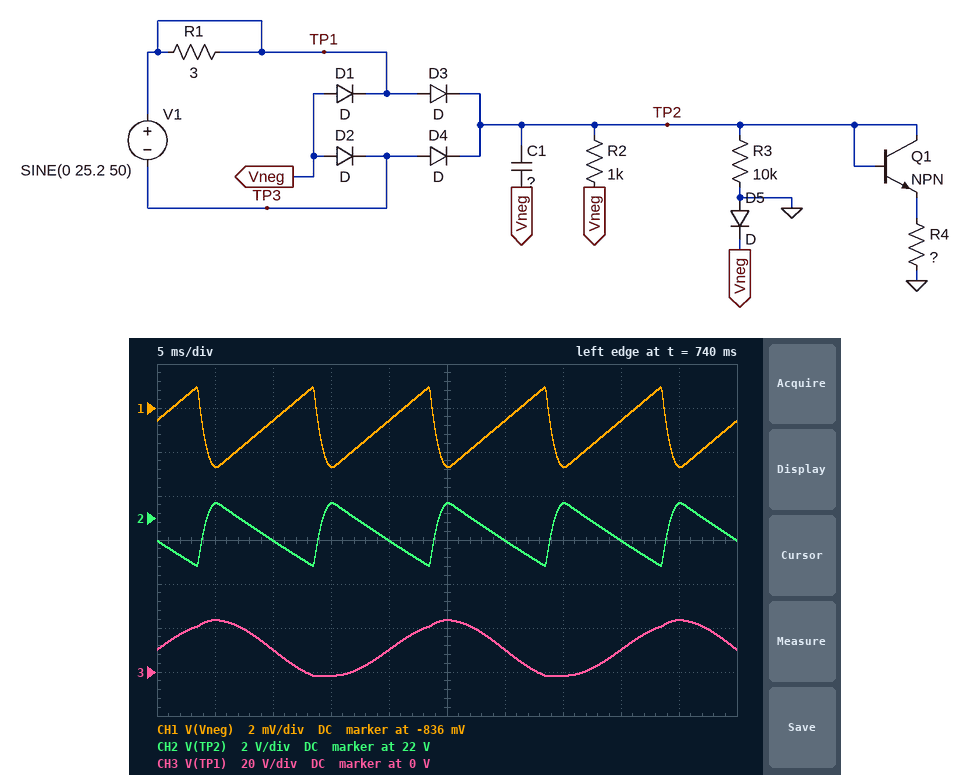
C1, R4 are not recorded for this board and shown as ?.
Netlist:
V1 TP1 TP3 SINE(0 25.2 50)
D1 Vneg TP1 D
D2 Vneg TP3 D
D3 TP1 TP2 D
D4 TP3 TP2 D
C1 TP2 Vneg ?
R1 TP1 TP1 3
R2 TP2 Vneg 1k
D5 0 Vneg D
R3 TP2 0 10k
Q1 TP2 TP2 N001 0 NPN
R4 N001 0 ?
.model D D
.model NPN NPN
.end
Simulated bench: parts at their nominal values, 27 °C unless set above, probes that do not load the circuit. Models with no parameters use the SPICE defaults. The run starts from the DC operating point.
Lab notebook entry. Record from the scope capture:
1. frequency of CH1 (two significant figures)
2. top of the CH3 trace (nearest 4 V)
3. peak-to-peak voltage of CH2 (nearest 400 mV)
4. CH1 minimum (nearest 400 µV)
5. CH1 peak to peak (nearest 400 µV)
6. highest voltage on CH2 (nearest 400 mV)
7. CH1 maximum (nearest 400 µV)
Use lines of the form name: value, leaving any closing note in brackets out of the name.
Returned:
frequency of CH1: 100 Hz
top of the CH3 trace: 24 V
peak-to-peak voltage of CH2: 2.8 V
CH1 minimum: -838.8 mV
CH1 peak to peak: 3.6 mV
highest voltage on CH2: 22.8 V
CH1 maximum: -835.2 mV
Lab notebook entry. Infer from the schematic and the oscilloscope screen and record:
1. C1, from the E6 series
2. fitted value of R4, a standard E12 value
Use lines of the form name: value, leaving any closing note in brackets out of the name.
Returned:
C1, from the E6 series: 3.3 mF
fitted value of R4, a standard E12 value: 18 Ω
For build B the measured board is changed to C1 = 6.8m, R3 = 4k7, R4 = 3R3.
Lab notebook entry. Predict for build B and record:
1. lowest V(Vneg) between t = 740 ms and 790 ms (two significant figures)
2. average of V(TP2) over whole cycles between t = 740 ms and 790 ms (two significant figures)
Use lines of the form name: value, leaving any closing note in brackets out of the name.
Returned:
lowest V(Vneg) between t = 740 ms and 790 ms: -880 mV
average of V(TP2) over whole cycles between t = 740 ms and 790 ms: 20 V
